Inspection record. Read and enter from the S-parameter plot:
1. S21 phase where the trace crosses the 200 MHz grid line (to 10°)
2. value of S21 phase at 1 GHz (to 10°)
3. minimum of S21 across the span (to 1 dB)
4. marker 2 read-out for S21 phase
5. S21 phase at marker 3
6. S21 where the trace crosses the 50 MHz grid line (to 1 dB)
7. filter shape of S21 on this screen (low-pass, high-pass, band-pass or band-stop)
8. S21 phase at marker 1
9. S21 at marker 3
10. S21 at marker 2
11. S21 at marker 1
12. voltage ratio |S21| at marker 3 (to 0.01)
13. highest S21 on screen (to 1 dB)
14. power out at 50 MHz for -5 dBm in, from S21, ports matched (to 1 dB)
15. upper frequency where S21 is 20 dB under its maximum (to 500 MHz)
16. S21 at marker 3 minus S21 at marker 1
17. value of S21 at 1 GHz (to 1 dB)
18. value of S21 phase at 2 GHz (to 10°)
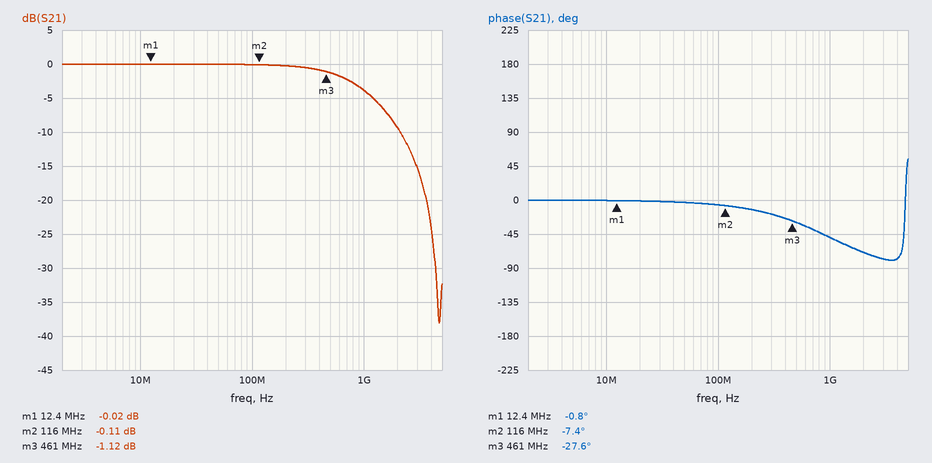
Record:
-10°
-50°
-38 dB
-7.4°
-27.6°
0 dB
low-pass
-0.8°
-1.12 dB
-0.11 dB
-0.02 dB
0.88
0 dB
-5 dBm
3.5 GHz
-1.10 dB
-4 dB
-70°
